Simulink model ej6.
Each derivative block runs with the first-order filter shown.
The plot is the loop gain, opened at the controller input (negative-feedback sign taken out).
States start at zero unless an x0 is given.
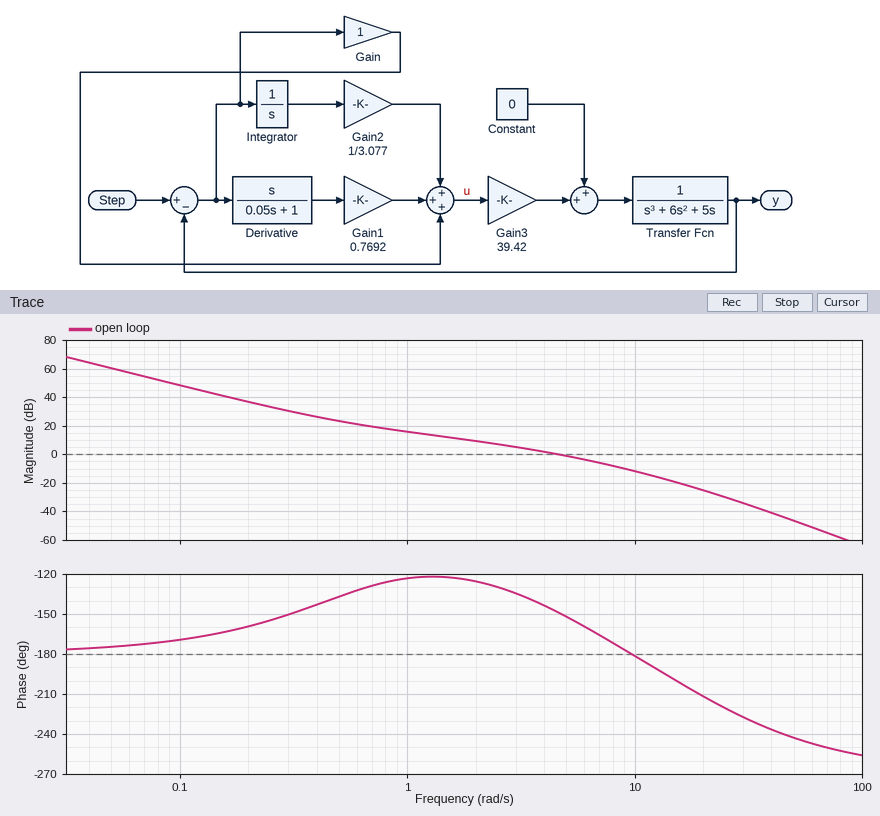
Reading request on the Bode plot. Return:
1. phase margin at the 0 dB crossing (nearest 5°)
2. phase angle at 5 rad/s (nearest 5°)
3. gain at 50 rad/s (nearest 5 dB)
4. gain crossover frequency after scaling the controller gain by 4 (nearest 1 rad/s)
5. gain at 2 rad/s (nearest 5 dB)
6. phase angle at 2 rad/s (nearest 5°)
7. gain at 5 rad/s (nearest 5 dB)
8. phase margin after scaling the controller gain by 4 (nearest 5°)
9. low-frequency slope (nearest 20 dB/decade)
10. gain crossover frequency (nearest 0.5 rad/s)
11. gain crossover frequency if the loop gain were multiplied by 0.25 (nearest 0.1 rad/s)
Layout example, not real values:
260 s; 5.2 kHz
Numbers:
30°; -150°; -45 dB; 10 rad/s; 10 dB; -125°; 0 dB; 0°; -40 dB/decade; 4.5 rad/s; 1.5 rad/s
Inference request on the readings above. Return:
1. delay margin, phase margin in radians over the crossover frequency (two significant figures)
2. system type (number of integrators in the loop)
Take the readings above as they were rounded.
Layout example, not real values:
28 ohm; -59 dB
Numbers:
0.12 s; 2
